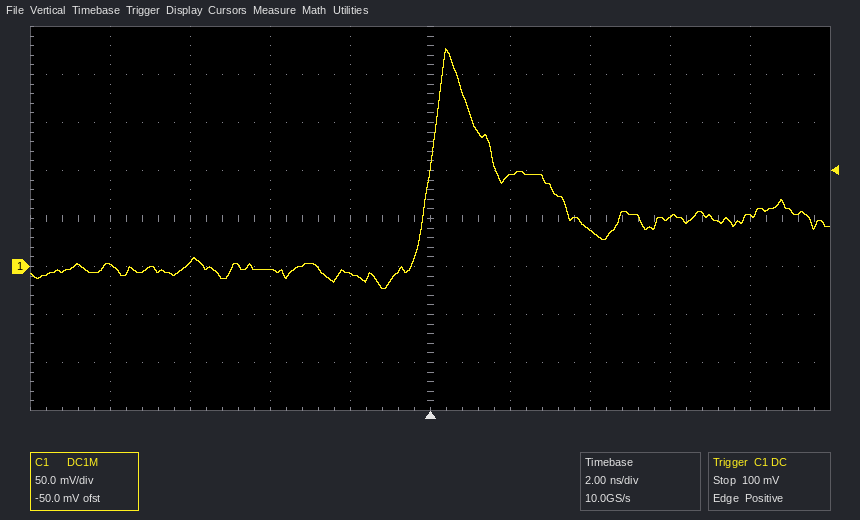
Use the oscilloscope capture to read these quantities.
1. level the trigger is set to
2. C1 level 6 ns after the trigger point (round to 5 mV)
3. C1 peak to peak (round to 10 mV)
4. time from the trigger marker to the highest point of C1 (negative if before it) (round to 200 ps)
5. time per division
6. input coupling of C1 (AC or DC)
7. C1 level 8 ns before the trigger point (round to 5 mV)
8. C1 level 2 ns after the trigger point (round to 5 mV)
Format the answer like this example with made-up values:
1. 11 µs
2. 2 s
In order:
1. 100 mV
2. 50 mV
3. 250 mV
4. +400 ps
5. 2 ns
6. DC
7. 0 mV
8. 95 mV
